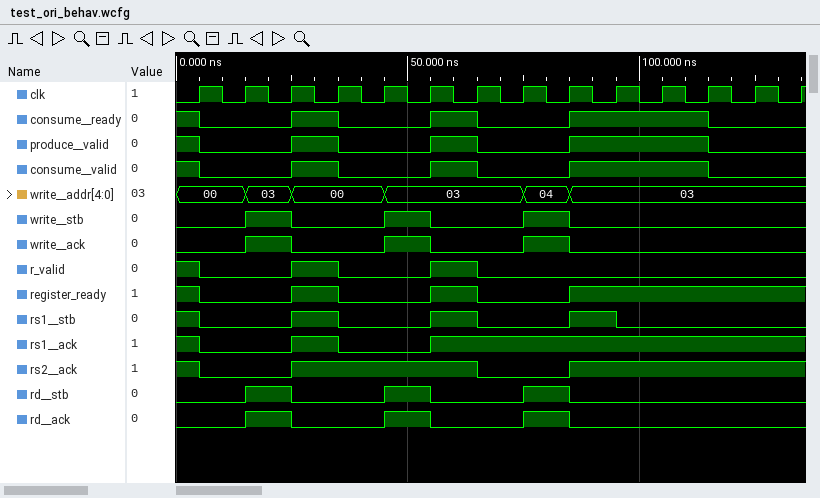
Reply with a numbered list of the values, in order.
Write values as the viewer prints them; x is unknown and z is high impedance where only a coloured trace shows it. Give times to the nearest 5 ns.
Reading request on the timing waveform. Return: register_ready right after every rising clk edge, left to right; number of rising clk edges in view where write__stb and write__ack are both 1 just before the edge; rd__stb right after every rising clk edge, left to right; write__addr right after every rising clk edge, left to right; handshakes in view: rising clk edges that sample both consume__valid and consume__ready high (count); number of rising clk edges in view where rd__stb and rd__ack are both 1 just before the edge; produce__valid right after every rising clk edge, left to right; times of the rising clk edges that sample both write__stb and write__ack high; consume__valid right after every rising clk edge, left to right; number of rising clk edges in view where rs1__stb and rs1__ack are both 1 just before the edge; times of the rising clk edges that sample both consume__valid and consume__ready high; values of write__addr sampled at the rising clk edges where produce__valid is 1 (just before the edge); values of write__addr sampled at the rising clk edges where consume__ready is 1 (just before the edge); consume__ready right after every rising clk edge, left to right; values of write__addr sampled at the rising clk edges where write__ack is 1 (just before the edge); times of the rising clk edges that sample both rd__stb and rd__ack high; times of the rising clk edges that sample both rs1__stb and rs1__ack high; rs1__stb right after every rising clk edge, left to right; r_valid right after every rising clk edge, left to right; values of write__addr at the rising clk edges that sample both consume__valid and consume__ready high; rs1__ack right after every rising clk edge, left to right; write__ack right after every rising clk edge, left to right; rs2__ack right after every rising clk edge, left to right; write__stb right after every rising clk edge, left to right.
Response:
1. 0 0 1 0 0 1 0 0 1 1 1 1 1 1
2. 3
3. 0 1 0 0 1 0 0 1 0 0 0 0 0 0
4. 00, 03, 00, 00, 03, 03, 03, 04, 03, 03, 03, 03, 03, 03
5. 6
6. 3
7. 0 0 1 0 0 1 0 0 1 1 1 0 0 0
8. 25 ns, 55 ns, 85 ns
9. 0 0 1 0 0 1 0 0 1 1 1 0 0 0
10. 4
11. 5 ns, 35 ns, 65 ns, 95 ns, 105 ns, 115 ns
12. 00, 00, 03, 03, 03, 03
13. 00, 00, 03, 03, 03, 03
14. 0 0 1 0 0 1 0 0 1 1 1 0 0 0
15. 03, 03, 04
16. 25 ns, 55 ns, 85 ns
17. 5 ns, 35 ns, 65 ns, 95 ns
18. 0 0 1 0 0 1 0 0 1 0 0 0 0 0
19. 0 0 1 0 0 1 0 0 0 0 0 0 0 0
20. 00, 00, 03, 03, 03, 03
21. 0 0 1 0 0 1 1 1 1 1 1 1 1 1
22. 0 1 0 0 1 0 0 1 0 0 0 0 0 0
23. 0 0 1 1 1 1 0 0 1 1 1 1 1 1
24. 0 1 0 0 1 0 0 1 0 0 0 0 0 0
